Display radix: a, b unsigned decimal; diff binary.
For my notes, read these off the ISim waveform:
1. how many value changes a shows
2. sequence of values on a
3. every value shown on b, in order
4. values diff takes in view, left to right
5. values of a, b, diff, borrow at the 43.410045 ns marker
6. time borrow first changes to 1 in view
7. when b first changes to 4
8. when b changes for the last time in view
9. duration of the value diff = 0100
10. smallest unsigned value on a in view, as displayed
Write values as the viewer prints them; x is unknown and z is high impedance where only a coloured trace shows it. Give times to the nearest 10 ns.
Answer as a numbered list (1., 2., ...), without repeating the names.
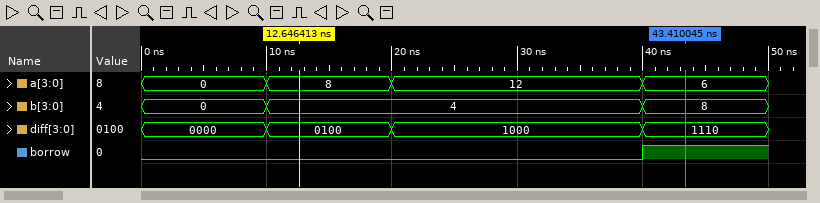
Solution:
1. 3
2. 0, 8, 12, 6
3. 0, 4, 8
4. 0000, 0100, 1000, 1110
5. a=6, b=8, diff=1110, borrow=1
6. 40 ns
7. 10 ns
8. 40 ns
9. 10 ns
10. 0
